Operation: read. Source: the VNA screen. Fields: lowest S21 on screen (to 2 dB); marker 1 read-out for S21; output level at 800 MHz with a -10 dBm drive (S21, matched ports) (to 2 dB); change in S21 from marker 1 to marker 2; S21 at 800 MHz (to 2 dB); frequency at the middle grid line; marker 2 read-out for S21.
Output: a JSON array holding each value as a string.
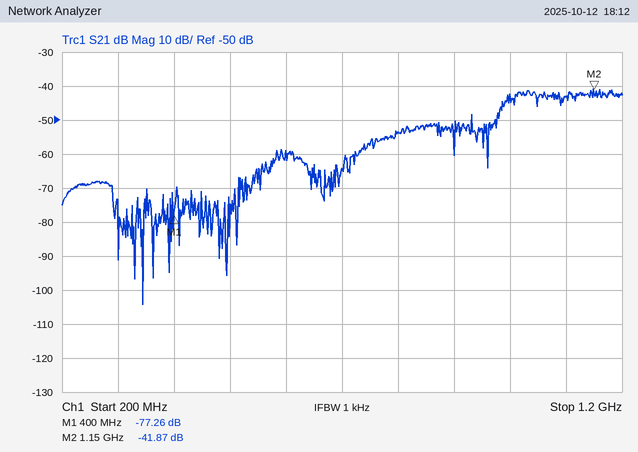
["-104 dB", "-77.26 dB", "-64 dBm", "35.39 dB", "-54 dB", "700 MHz", "-41.87 dB"]
